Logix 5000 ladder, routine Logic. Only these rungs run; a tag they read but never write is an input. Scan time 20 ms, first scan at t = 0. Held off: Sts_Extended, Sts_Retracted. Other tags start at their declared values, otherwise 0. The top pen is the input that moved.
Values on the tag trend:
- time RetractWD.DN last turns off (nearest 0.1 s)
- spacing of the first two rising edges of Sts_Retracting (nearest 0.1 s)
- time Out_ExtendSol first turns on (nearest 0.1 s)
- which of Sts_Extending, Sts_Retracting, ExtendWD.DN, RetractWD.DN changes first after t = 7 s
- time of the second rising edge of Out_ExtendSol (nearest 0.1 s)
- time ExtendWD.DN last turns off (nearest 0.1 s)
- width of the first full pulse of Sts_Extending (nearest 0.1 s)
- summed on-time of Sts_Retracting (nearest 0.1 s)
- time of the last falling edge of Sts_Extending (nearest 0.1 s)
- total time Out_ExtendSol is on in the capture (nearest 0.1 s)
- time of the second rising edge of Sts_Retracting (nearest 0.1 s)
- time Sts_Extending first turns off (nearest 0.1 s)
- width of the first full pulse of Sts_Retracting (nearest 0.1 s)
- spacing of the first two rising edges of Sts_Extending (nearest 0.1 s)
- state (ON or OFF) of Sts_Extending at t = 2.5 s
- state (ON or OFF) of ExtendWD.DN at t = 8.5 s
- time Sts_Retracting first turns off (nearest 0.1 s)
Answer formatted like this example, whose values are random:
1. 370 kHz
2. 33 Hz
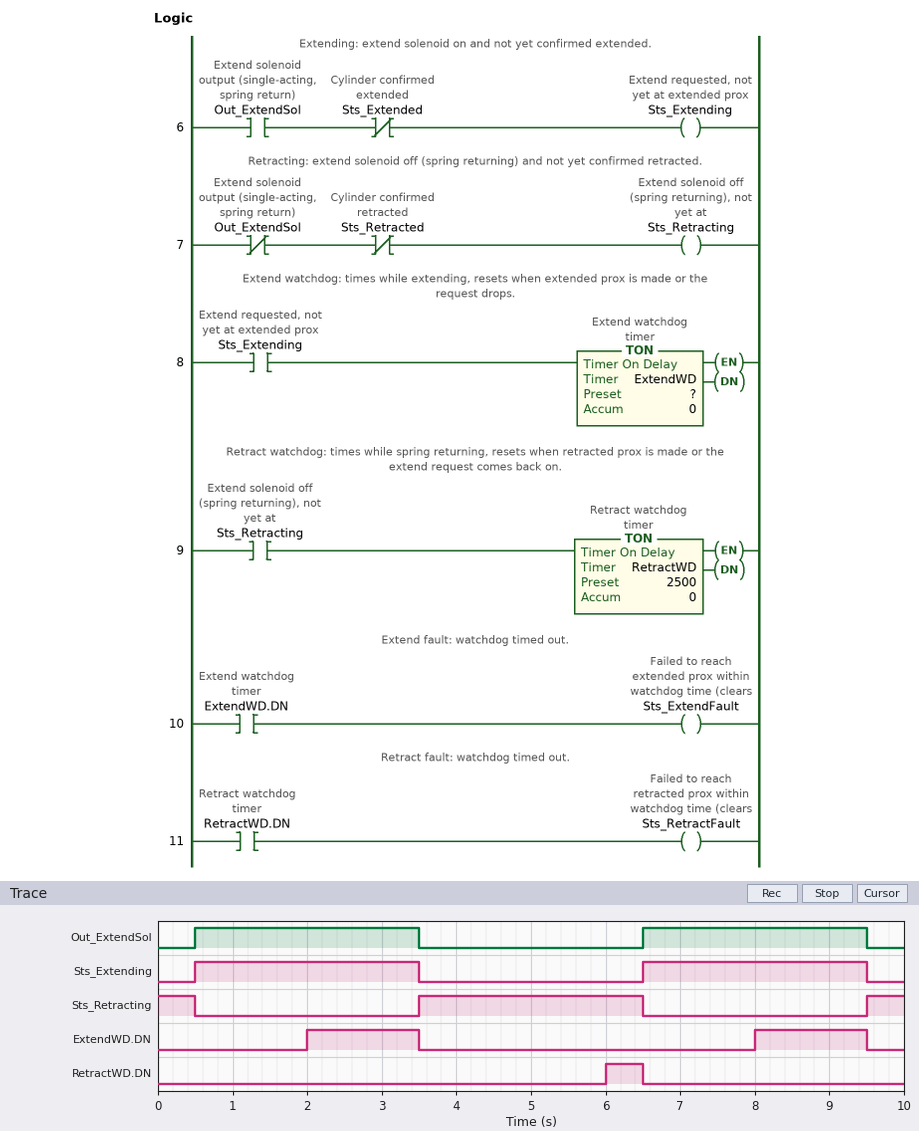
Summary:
1. 6.5 s
2. 6.0 s
3. 0.5 s
4. ExtendWD.DN
5. 6.5 s
6. 9.5 s
7. 3.0 s
8. 4.0 s
9. 9.5 s
10. 6.0 s
11. 9.5 s
12. 3.5 s
13. 3.0 s
14. 6.0 s
15. ON
16. ON
17. 0.5 s
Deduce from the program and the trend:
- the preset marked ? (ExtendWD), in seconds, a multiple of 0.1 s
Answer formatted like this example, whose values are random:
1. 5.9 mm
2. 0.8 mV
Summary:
1. 1.5 s
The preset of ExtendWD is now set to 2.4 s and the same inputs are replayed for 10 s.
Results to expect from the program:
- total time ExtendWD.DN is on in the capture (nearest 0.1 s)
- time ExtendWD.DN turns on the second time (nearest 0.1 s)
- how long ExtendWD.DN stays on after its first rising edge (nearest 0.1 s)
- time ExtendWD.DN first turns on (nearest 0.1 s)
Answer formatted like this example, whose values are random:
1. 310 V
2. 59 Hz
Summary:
1. 1.2 s
2. 8.9 s
3. 0.6 s
4. 2.9 s
